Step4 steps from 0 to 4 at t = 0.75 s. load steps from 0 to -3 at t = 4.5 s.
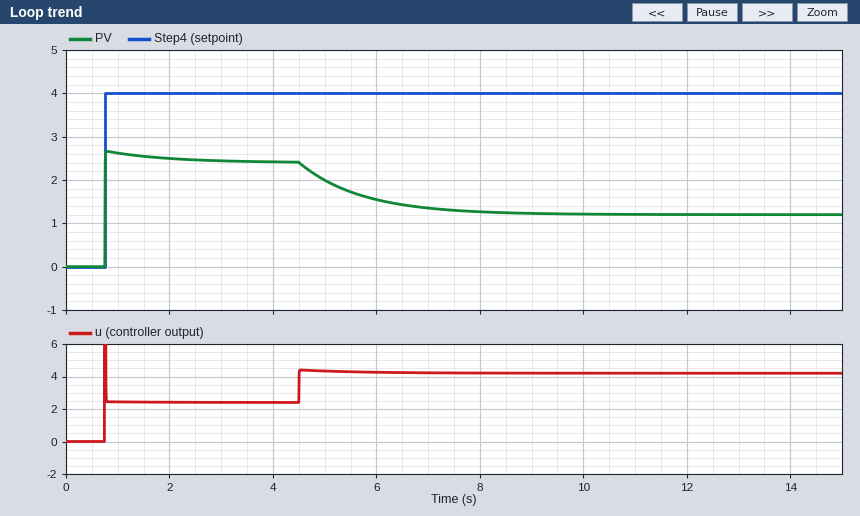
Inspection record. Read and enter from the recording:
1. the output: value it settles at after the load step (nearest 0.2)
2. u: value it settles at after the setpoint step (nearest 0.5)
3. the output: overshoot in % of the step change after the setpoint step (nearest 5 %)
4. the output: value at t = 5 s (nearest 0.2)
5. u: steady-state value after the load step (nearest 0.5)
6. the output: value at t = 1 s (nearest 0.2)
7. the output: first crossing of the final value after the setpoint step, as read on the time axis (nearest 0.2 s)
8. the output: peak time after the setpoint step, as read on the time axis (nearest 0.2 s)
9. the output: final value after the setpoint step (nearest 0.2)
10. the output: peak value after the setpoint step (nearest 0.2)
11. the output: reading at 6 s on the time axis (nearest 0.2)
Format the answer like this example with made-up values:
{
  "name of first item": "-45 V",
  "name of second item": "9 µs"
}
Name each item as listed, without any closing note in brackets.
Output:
{
  "the output: value it settles at after the load step": "1.2",
  "u: value it settles at after the setpoint step": "2.5",
  "the output: overshoot in % of the step change after the setpoint step": "10 %",
  "the output: value at t = 5 s": "2.0",
  "u: steady-state value after the load step": "4.0",
  "the output: value at t = 1 s": "2.6",
  "the output: first crossing of the final value after the setpoint step, as read on the time axis": "0.8 s",
  "the output: peak time after the setpoint step, as read on the time axis": "0.8 s",
  "the output: final value after the setpoint step": "2.4",
  "the output: peak value after the setpoint step": "2.6",
  "the output: reading at 6 s on the time axis": "1.6"
}
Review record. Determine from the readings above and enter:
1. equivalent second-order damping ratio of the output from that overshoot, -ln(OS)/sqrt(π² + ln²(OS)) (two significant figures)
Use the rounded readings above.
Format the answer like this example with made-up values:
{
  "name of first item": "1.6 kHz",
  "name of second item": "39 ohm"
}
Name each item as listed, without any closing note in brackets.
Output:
{
  "equivalent second-order damping ratio of the output from that overshoot, -ln(OS)/sqrt(π² + ln²(OS))": "0.59"
}
